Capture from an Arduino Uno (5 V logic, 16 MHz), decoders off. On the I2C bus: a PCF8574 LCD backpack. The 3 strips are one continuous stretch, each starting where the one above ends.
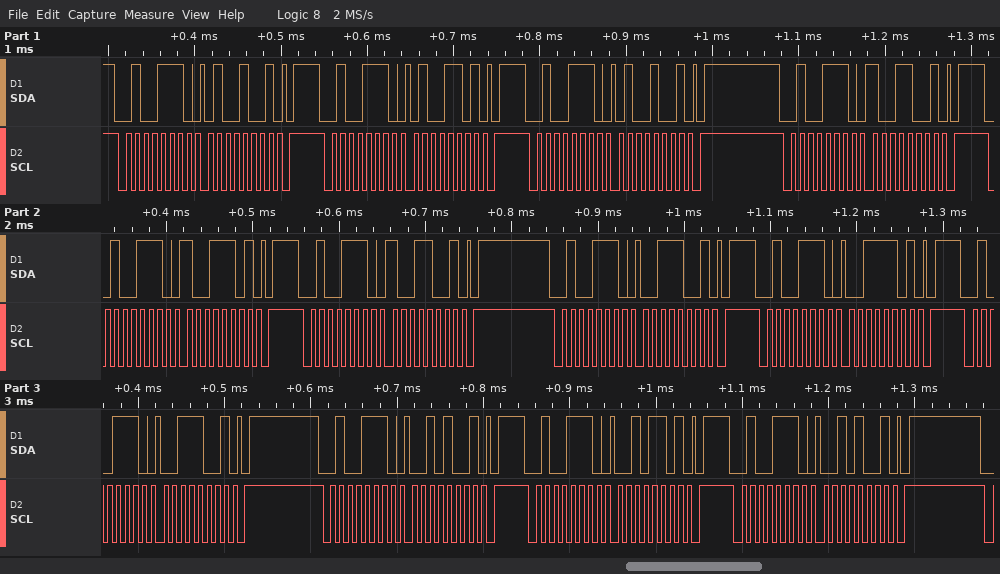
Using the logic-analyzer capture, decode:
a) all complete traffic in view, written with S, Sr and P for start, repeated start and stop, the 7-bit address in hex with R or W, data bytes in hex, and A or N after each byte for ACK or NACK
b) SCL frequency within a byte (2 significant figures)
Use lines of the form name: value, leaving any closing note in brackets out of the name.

all complete traffic in view, written with S, Sr and P for start, repeated start and stop, the 7-bit address in hex with R or W, data bytes in hex, and A or N after each byte for ACK or NACK: S 27W A 49 A P S 27W A 4D A P S 27W A 49 A P S 27W A 99 A P S 27W A 9D A P S 27W A 99 A P S 27W A 39 A P S 27W A 3D A P S 27W A 39 A P S 27W A 29 A P S 27W A 2D A P S 27W A 29 A P
SCL frequency within a byte: 100 kHz
